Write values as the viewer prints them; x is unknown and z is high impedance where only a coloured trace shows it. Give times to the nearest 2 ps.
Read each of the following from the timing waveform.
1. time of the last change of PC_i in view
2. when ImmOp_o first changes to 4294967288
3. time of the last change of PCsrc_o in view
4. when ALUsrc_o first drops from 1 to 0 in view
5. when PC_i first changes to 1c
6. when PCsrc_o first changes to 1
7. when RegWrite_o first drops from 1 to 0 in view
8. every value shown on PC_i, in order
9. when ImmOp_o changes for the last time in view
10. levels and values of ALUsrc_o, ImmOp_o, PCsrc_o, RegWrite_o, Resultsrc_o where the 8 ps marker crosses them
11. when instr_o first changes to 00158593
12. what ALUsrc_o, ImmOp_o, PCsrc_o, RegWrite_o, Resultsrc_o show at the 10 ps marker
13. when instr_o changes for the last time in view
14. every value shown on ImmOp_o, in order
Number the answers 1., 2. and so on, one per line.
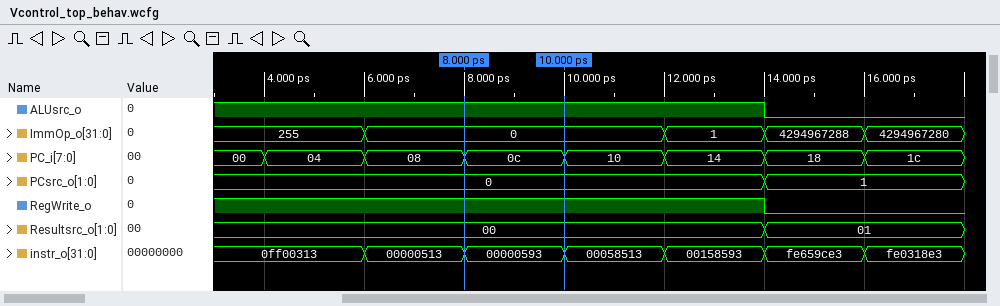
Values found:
1. 16 ps
2. 14 ps
3. 14 ps
4. 14 ps
5. 16 ps
6. 14 ps
7. 14 ps
8. 00, 04, 08, 0c, 10, 14, 18, 1c
9. 16 ps
10. ALUsrc_o=1, ImmOp_o=0, PCsrc_o=0, RegWrite_o=1, Resultsrc_o=00
11. 12 ps
12. ALUsrc_o=1, ImmOp_o=0, PCsrc_o=0, RegWrite_o=1, Resultsrc_o=00
13. 16 ps
14. 255, 0, 1, 4294967288, 4294967280
